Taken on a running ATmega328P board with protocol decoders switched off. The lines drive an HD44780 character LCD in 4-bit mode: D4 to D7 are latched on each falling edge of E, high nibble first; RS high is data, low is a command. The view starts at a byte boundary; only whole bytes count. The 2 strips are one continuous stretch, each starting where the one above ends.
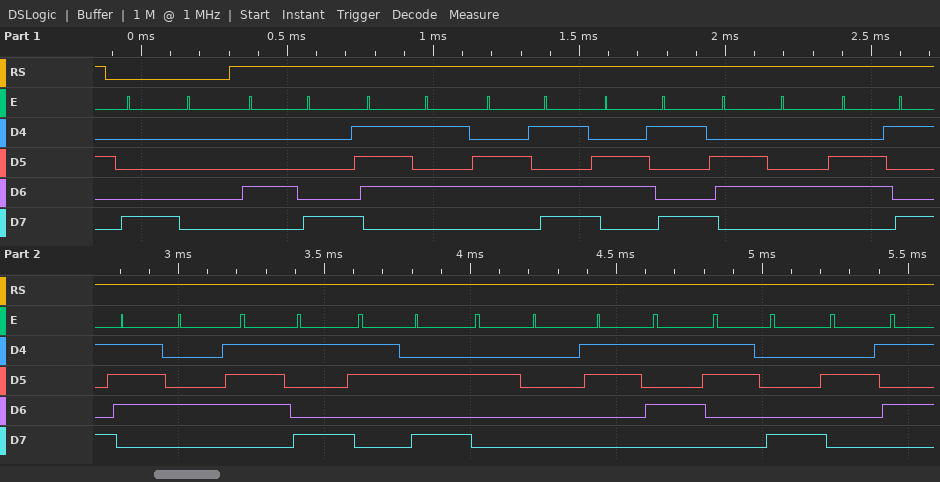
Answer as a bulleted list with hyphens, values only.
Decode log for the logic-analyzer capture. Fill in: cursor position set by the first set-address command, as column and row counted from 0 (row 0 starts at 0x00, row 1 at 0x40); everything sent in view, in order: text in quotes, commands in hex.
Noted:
- column 0, row 0
- 0x80 "Humidity: 58%"
